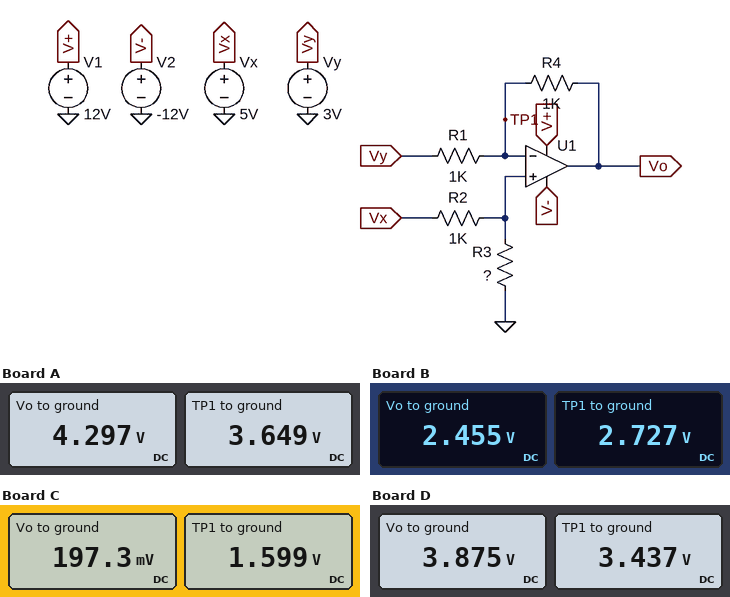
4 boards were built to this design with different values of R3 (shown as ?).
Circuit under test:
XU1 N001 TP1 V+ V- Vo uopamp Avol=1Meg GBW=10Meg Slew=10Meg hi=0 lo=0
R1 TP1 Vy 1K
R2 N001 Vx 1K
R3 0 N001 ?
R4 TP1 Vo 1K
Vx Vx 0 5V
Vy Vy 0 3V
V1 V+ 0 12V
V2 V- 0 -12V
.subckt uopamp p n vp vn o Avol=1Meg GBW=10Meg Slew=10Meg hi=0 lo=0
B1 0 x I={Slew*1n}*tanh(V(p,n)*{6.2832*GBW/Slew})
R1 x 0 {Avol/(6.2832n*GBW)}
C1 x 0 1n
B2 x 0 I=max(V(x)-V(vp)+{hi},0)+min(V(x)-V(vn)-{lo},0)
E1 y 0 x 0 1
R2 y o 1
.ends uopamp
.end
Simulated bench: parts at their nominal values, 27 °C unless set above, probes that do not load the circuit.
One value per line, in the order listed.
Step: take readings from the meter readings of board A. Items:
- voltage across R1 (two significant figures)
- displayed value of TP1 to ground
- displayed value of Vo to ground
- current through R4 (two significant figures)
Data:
650 mV
3.649 V
4.297 V
650 µA
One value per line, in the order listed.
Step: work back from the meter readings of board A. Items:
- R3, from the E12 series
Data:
2.7 kΩ
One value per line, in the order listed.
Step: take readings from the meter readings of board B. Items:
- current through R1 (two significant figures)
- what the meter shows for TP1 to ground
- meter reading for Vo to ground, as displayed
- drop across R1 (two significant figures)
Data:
270 µA
2.727 V
2.455 V
270 mV
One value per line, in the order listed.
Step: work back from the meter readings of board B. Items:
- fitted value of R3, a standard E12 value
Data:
1.2 kΩ
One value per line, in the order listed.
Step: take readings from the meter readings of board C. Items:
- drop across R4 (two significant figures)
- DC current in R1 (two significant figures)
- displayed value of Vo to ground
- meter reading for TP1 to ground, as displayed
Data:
1.4 V
1.4 mA
197.3 mV
1.599 V
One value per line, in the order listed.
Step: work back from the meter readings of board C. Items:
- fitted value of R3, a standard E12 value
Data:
470 Ω
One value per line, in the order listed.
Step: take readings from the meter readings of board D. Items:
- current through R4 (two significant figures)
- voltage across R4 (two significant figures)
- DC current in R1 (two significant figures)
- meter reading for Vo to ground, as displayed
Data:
440 µA
440 mV
440 µA
3.875 V
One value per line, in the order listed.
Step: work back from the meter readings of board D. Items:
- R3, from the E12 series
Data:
2.2 kΩ
